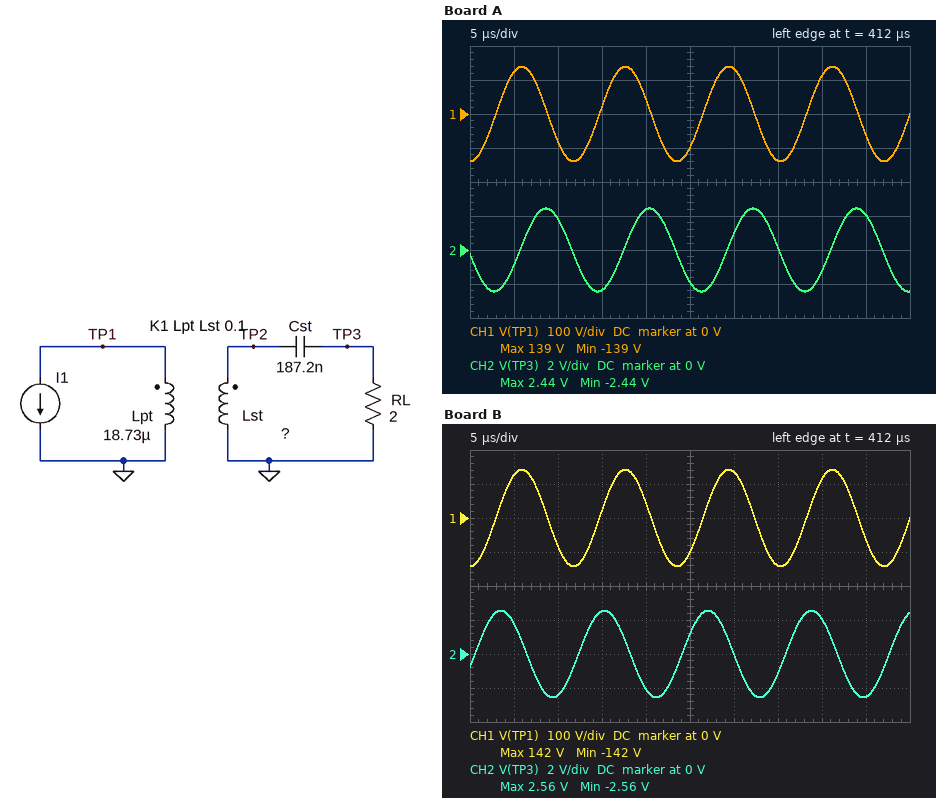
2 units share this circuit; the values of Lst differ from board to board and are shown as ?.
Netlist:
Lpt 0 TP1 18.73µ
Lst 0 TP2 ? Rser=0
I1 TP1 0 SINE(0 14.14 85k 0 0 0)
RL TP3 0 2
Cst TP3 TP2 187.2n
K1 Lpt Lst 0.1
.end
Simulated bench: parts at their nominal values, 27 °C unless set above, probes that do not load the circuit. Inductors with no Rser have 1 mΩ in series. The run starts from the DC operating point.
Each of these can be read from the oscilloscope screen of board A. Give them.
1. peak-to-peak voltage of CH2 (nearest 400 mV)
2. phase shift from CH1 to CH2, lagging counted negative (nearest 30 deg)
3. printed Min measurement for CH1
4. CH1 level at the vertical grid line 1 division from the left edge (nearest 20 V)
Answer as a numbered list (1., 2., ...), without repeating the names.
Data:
1. 4.8 V
2. -90 deg
3. -139 V
4. 120 V
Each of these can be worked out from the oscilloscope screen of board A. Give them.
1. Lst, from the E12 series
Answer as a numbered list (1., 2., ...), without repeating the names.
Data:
1. 56 µH
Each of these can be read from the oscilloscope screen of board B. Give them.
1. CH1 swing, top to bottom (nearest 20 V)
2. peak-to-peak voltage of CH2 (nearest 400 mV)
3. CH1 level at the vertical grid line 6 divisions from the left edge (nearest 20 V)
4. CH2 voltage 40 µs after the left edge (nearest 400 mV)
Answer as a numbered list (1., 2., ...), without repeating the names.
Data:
1. 280 V
2. 5.2 V
3. 140 V
4. 2.0 V
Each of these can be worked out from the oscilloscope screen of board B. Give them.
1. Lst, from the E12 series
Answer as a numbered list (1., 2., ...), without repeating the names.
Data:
1. 6.8 µH
